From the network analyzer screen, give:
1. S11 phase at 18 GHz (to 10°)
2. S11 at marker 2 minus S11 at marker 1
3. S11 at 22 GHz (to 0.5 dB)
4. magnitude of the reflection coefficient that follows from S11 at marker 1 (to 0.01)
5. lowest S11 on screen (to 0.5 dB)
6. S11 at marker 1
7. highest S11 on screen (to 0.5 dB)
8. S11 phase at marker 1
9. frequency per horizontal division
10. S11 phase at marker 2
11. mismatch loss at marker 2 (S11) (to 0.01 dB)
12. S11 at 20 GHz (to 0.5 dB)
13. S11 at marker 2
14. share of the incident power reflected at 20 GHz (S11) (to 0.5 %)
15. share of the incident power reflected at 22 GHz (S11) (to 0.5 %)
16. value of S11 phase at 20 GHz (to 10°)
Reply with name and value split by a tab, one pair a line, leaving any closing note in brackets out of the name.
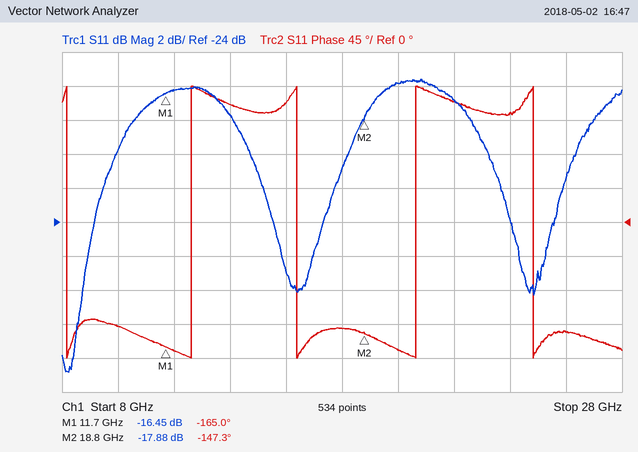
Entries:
S11 phase at 18 GHz	-140°
S11 at marker 2 minus S11 at marker 1	-1.43 dB
S11 at 22 GHz	-17.0 dB
magnitude of the reflection coefficient that follows from S11 at marker 1	0.15
lowest S11 on screen	-33.0 dB
S11 at marker 1	-16.45 dB
highest S11 on screen	-15.5 dB
S11 phase at marker 1	-165.0°
frequency per horizontal division	2 GHz
S11 phase at marker 2	-147.3°
mismatch loss at marker 2 (S11)	0.07 dB
S11 at 20 GHz	-16.0 dB
S11 at marker 2	-17.88 dB
share of the incident power reflected at 20 GHz (S11)	2.5 %
share of the incident power reflected at 22 GHz (S11)	2.0 %
value of S11 phase at 20 GHz	-170°
